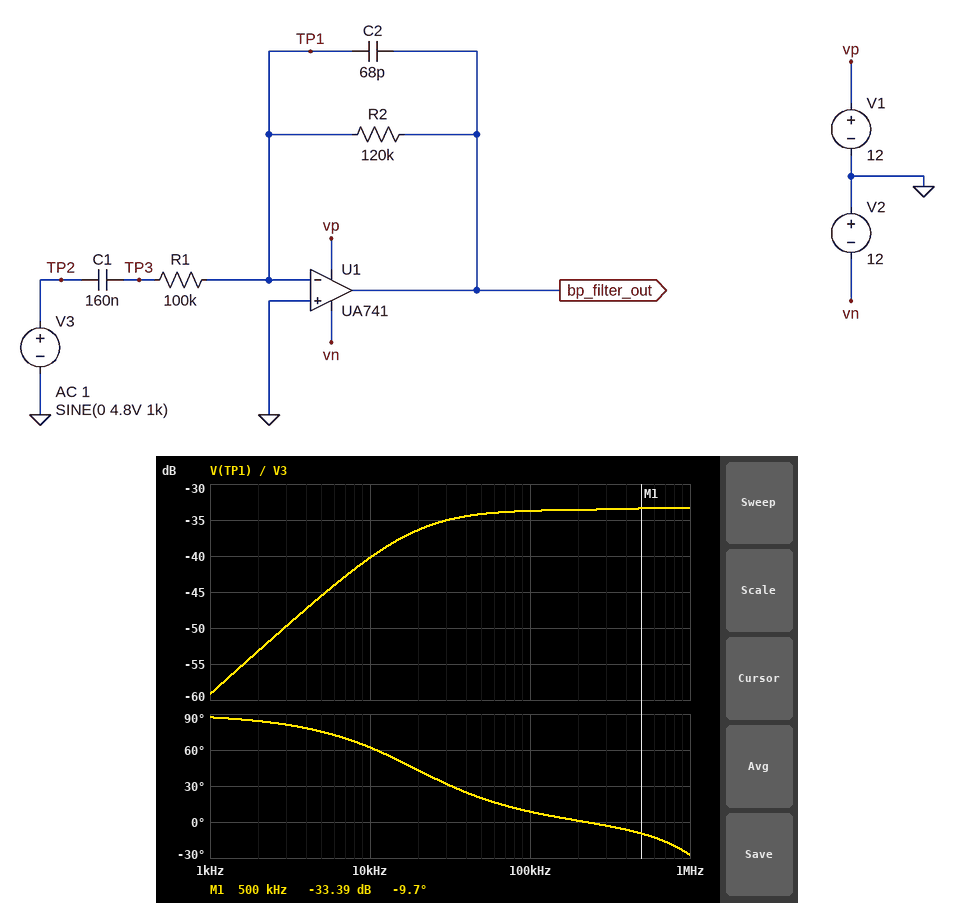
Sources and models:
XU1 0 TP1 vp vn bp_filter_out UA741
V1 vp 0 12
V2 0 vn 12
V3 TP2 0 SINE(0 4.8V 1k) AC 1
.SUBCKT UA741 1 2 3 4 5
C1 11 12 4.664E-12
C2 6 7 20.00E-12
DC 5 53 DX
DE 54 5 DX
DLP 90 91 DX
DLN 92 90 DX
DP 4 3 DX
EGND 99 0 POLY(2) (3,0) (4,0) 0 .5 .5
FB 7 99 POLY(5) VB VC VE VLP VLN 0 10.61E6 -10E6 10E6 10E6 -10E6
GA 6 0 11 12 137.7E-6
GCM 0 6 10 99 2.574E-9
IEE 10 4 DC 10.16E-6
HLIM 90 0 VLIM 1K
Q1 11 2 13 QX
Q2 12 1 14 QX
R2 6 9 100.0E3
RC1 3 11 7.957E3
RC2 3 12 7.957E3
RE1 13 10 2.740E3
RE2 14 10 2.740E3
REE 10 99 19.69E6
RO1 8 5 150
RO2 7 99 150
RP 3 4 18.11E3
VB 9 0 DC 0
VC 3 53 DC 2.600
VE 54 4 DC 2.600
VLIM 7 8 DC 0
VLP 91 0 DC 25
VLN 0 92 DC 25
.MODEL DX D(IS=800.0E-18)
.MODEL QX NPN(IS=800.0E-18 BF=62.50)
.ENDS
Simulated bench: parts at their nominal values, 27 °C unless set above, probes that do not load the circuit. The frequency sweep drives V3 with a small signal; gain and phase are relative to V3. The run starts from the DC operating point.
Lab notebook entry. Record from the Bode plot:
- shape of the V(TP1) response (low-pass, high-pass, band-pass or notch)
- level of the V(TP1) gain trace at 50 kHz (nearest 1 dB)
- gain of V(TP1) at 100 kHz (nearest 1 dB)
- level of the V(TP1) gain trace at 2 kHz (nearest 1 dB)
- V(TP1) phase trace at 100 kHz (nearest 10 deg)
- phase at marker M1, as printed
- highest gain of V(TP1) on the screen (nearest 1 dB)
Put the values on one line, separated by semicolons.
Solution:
high-pass; -34 dB; -34 dB; -53 dB; 10 deg; -9.7 deg; -33 dB
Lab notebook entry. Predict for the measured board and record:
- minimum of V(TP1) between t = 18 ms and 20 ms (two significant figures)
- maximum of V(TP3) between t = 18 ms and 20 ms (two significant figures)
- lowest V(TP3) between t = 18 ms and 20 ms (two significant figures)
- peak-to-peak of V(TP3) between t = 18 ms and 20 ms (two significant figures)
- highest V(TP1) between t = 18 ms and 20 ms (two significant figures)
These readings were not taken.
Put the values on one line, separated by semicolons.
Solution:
-5.3 mV; 4.8 V; -4.8 V; 9.6 V; 5.3 mV
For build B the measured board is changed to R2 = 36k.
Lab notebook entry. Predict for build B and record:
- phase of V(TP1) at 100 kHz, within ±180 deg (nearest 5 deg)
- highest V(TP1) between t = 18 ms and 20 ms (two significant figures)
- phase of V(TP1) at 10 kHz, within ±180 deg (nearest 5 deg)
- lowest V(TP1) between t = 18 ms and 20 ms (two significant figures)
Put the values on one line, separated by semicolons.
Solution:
30 deg; 1.6 mV; 80 deg; -1.6 mV
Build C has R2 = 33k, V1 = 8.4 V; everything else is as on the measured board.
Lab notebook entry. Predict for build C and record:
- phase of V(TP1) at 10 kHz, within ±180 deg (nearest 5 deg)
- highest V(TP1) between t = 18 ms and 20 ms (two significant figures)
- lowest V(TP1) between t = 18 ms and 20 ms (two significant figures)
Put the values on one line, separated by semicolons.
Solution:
80 deg; 1.4 mV; -1.5 mV
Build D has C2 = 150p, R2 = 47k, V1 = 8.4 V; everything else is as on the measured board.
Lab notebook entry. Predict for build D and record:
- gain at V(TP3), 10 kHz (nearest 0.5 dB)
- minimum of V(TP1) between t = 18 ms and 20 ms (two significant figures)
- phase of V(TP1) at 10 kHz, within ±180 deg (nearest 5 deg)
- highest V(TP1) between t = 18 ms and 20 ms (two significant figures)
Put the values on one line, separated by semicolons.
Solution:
0 dB; -2.1 mV; 65 deg; 2.0 mV
